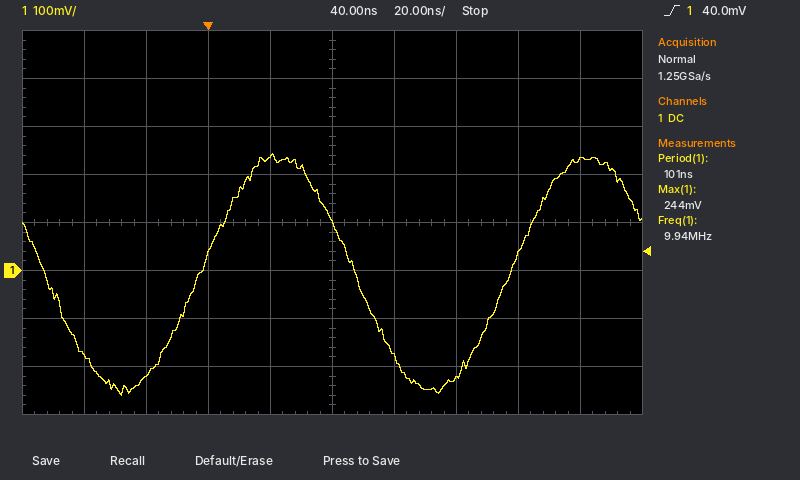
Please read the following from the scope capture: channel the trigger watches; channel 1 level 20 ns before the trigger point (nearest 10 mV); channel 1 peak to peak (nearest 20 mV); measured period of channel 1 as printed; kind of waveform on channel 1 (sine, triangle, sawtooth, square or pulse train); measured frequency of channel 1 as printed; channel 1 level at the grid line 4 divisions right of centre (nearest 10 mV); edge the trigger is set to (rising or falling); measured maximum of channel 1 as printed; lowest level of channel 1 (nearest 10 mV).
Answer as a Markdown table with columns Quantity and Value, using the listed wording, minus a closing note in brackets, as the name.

| Quantity | Value |
|---|---|
| channel the trigger watches | channel 1 |
| channel 1 level 20 ns before the trigger point | -220 mV |
| channel 1 peak to peak | 500 mV |
| measured period of channel 1 as printed | 101 ns |
| kind of waveform on channel 1 | sine |
| measured frequency of channel 1 as printed | 9.94 MHz |
| channel 1 level at the grid line 4 divisions right of centre | 230 mV |
| edge the trigger is set to | rising |
| measured maximum of channel 1 as printed | 244 mV |
| lowest level of channel 1 | -260 mV |
